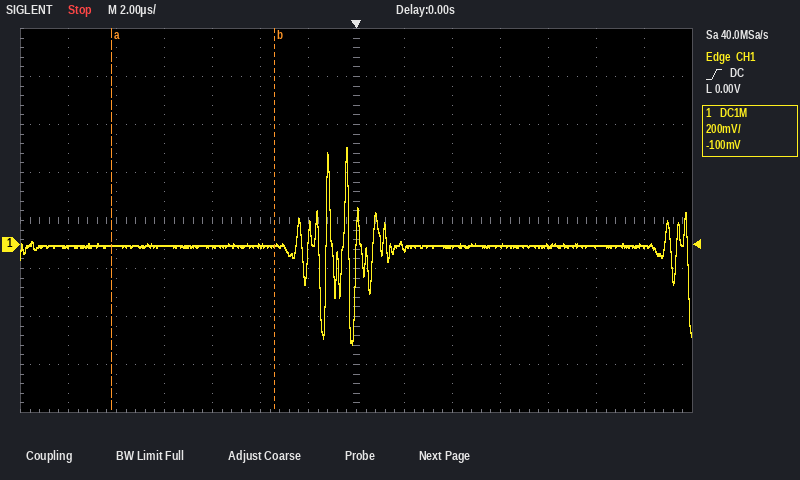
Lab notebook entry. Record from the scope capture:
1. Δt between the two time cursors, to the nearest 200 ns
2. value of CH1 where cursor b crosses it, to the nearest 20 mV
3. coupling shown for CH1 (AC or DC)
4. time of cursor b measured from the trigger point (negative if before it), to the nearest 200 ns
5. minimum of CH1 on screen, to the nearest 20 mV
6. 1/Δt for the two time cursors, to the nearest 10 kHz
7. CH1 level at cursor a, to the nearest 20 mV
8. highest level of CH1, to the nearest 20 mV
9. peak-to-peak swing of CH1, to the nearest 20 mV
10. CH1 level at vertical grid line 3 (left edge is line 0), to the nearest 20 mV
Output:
6.8 µs
0 mV
DC
-3.4 µs
-420 mV
150 kHz
0 mV
400 mV
820 mV
0 mV
